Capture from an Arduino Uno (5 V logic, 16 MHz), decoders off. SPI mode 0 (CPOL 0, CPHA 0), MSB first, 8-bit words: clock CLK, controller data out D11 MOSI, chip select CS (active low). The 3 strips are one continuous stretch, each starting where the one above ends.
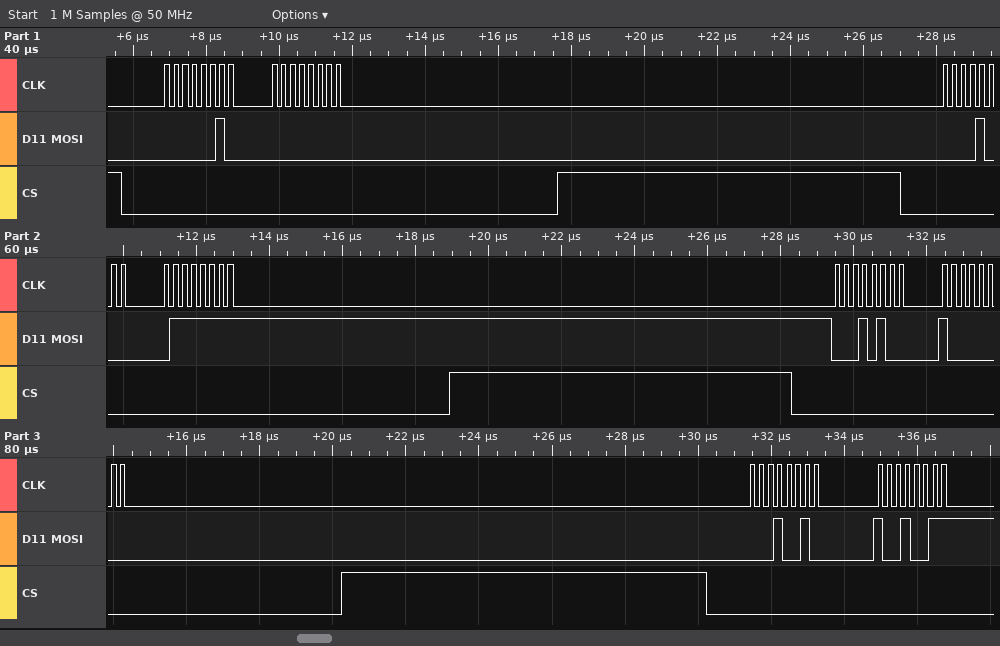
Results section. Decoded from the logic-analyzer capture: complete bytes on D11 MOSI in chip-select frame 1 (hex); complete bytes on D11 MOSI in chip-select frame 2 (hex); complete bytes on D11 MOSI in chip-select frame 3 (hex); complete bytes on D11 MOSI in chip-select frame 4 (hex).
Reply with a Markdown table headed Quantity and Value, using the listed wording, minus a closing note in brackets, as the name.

| Quantity | Value |
|---|---|
| complete bytes on D11 MOSI in chip-select frame 1 | 02 00 |
| complete bytes on D11 MOSI in chip-select frame 2 | 08 7F |
| complete bytes on D11 MOSI in chip-select frame 3 | 14 80 |
| complete bytes on D11 MOSI in chip-select frame 4 | 12 93 |
